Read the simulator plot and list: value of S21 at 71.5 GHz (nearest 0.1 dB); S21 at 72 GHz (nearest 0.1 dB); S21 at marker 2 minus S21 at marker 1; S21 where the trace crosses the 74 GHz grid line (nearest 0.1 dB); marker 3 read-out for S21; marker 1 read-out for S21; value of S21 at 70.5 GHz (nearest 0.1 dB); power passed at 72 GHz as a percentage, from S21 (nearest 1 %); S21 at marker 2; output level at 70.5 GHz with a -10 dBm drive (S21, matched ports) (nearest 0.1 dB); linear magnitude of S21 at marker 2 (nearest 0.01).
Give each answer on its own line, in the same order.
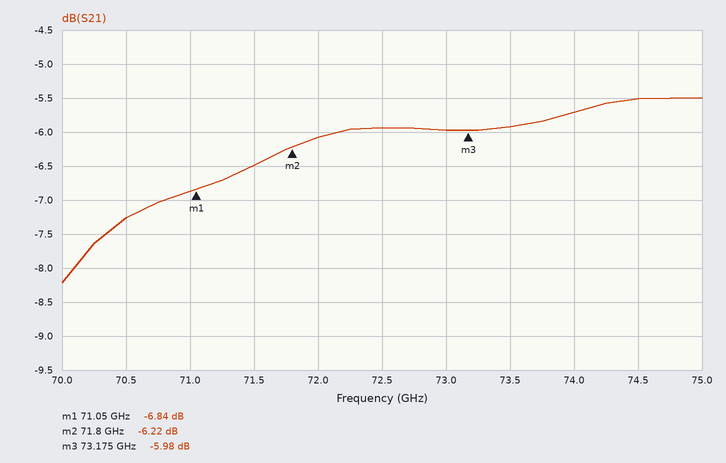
-6.5 dB
-6.1 dB
0.62 dB
-5.7 dB
-5.98 dB
-6.84 dB
-7.3 dB
25 %
-6.22 dB
-17.3 dBm
0.49
